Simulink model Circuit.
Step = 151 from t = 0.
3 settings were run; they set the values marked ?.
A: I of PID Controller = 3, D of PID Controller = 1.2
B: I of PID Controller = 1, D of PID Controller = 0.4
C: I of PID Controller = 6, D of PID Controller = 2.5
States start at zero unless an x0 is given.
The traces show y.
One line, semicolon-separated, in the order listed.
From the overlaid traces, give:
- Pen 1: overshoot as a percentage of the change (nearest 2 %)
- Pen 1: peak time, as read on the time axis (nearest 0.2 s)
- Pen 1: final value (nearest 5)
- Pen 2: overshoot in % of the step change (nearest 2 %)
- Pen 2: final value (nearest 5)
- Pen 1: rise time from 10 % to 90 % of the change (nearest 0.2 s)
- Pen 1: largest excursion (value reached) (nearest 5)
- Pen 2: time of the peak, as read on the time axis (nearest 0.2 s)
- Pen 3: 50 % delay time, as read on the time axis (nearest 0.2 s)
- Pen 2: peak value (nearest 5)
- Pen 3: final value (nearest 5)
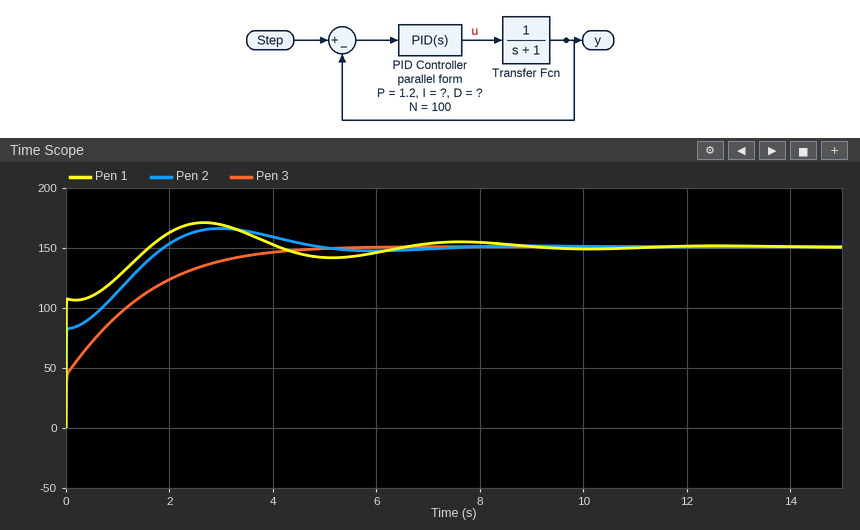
14 %; 2.6 s; 150; 10 %; 150; 1.2 s; 170; 3.0 s; 0.6 s; 165; 150
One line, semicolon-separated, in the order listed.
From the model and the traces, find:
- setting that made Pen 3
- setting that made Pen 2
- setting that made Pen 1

B; A; C
